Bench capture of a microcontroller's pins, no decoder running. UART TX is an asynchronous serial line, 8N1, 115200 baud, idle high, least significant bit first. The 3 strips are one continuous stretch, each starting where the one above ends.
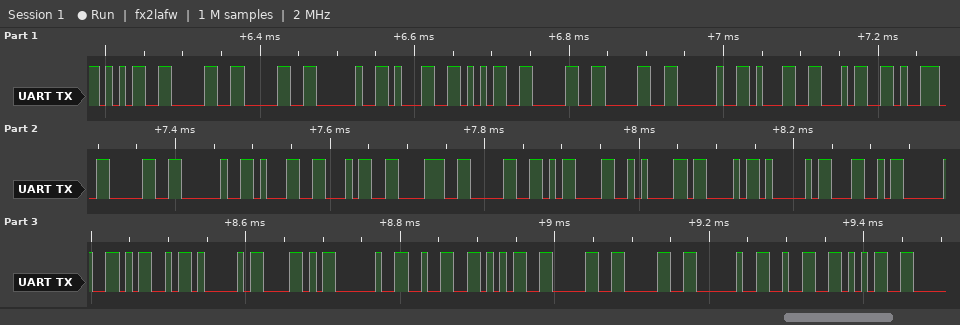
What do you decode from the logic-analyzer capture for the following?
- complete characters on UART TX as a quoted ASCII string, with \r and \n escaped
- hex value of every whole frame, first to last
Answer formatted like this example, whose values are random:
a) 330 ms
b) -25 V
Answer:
a) "500 1500 1490 1480\r\nCAL MAX 2500 25"
b) 35 30 30 20 31 35 30 30 20 31 34 39 30 20 31 34 38 30 0D 0A 43 41 4C 20 4D 41 58 20 32 35 30 30 20 32 35
